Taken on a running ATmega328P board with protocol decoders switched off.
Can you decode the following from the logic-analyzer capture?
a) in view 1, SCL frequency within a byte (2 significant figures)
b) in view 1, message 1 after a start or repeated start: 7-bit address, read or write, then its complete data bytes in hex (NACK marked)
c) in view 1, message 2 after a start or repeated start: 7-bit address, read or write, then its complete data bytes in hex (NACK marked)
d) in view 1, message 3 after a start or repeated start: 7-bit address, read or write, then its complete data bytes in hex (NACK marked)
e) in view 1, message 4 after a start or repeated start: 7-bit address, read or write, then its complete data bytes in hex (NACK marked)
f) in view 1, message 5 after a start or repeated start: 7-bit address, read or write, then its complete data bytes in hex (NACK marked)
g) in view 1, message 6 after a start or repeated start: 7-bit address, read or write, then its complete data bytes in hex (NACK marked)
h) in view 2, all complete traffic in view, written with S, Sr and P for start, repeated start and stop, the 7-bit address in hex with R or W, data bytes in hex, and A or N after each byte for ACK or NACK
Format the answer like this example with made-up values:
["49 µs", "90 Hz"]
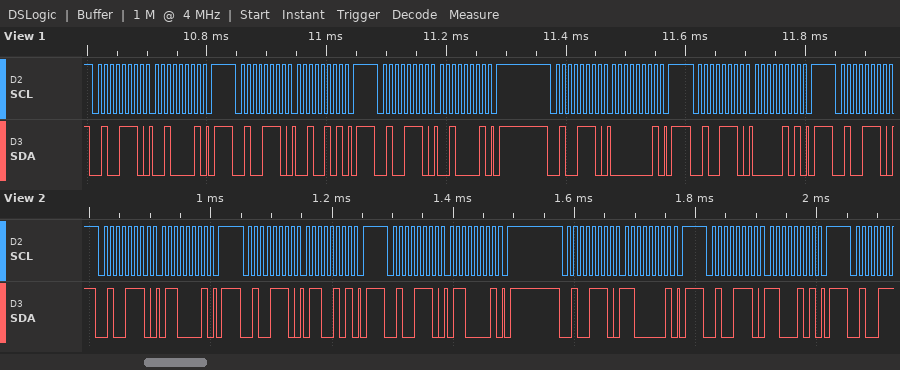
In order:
["100 kHz", "0x27 write: 21", "0x27 write: 25", "0x27 write: 21", "0x27 write: 01", "0x27 write: 05", "0x27 write", "S 27W A 61 A P S 27W A 65 A P S 27W A 61 A P S 27W A C1 A P S 27W A C5 A P"]
